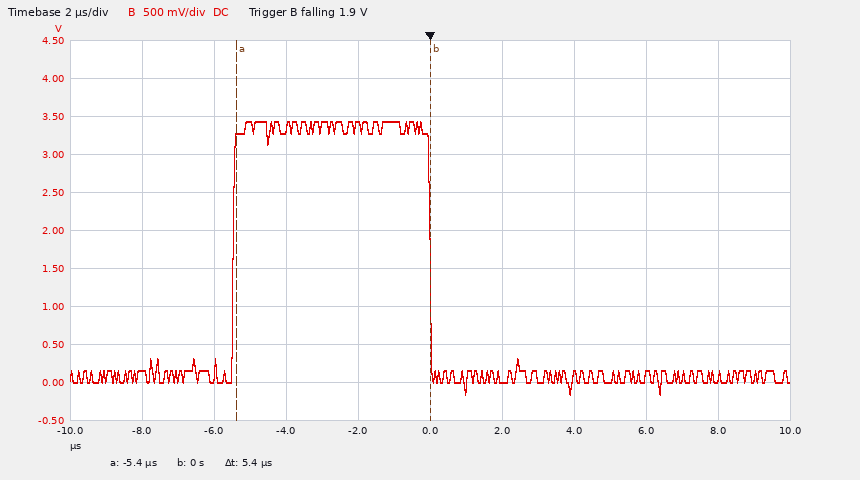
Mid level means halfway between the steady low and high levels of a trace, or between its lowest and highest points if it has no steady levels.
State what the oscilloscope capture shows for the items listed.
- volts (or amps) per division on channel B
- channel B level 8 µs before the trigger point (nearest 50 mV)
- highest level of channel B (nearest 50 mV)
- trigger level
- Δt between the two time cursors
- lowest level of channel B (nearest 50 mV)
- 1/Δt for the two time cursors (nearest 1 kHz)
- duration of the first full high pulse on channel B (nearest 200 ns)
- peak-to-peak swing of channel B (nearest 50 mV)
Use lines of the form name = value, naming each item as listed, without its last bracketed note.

volts (or amps) per division on channel B = 500 mV
channel B level 8 µs before the trigger point = 150 mV
highest level of channel B = 3.45 V
trigger level = 1.9 V
Δt between the two time cursors = 5.4 µs
lowest level of channel B = -150 mV
1/Δt for the two time cursors = 185 kHz
duration of the first full high pulse on channel B = 5.4 µs
peak-to-peak swing of channel B = 3.60 V
